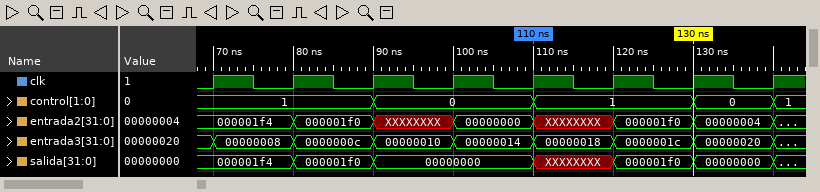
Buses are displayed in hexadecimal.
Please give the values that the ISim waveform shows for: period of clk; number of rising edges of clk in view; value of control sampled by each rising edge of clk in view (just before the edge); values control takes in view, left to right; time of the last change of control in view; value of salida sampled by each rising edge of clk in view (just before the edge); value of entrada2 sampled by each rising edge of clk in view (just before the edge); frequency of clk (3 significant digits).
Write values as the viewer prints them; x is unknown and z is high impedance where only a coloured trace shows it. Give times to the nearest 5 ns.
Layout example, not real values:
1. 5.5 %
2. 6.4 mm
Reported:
1. 10 ns
2. 8
3. 1, 1, 1, 0, 0, 1, 1, 0
4. 1, 0, 1, 0, 1
5. 140 ns
6. 000001f4, 000001f4, 000001f0, 00000000, 00000000, XXXXXXXX, 000001f0, 00000000
7. 000001f4, 000001f4, 000001f0, XXXXXXXX, 00000000, XXXXXXXX, 000001f0, 00000004
8. 100 MHz
